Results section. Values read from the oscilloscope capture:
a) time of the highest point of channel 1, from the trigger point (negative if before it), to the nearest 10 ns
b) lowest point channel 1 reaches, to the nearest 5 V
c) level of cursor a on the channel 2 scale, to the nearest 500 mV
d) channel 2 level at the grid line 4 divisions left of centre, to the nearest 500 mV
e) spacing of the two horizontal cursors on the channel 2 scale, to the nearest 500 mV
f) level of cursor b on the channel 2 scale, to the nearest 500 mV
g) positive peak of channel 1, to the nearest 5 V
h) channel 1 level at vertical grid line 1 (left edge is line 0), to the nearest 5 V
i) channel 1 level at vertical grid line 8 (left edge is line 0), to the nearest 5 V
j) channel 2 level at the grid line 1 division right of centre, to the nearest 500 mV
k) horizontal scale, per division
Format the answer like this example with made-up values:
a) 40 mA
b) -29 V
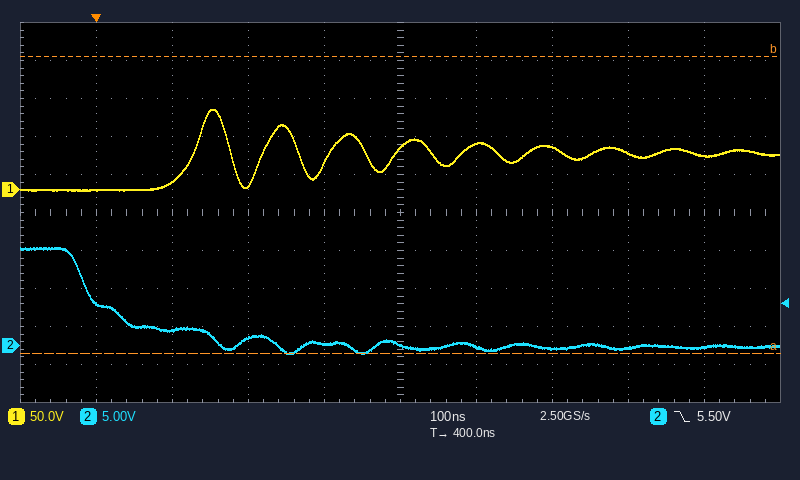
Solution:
a) +150 ns
b) 0 V
c) -1.0 V
d) 5.5 V
e) 39.0 V
f) 38.0 V
g) 105 V
h) 0 V
i) 50 V
j) 0.0 V
k) 100 ns
